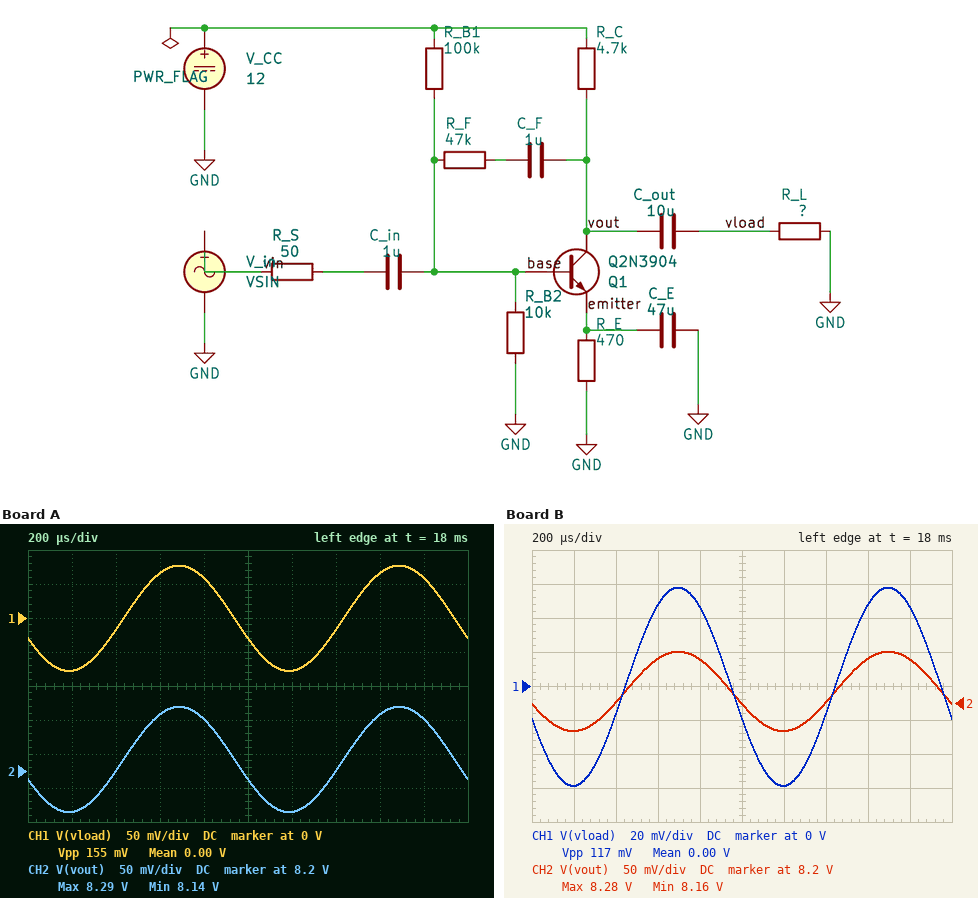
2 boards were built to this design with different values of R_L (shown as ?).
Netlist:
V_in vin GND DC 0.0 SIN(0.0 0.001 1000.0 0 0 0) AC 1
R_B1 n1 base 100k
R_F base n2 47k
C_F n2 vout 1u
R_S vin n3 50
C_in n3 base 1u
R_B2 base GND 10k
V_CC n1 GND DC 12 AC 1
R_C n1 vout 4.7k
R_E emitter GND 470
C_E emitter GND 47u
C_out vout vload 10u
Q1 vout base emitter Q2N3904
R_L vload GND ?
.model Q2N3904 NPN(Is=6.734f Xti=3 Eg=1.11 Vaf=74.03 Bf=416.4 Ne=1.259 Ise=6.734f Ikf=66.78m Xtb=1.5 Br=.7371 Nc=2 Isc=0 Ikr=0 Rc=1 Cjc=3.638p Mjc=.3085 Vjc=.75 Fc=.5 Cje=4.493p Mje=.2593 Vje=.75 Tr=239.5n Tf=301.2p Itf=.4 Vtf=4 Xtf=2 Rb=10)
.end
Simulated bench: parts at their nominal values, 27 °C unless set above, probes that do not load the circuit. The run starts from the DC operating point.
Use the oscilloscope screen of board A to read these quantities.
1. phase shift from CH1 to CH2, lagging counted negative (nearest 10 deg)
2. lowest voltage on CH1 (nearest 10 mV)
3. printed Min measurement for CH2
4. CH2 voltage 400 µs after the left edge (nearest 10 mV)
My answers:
0 deg
-80 mV
8.14 V
8.20 V
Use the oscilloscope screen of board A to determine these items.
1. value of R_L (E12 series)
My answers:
12 kΩ
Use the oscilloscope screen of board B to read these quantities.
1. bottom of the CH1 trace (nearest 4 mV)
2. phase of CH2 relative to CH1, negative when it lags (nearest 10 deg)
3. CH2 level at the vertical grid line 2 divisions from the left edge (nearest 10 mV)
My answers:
-60 mV
0 deg
8.20 V
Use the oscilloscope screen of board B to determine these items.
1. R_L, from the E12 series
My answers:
4.7 kΩ
